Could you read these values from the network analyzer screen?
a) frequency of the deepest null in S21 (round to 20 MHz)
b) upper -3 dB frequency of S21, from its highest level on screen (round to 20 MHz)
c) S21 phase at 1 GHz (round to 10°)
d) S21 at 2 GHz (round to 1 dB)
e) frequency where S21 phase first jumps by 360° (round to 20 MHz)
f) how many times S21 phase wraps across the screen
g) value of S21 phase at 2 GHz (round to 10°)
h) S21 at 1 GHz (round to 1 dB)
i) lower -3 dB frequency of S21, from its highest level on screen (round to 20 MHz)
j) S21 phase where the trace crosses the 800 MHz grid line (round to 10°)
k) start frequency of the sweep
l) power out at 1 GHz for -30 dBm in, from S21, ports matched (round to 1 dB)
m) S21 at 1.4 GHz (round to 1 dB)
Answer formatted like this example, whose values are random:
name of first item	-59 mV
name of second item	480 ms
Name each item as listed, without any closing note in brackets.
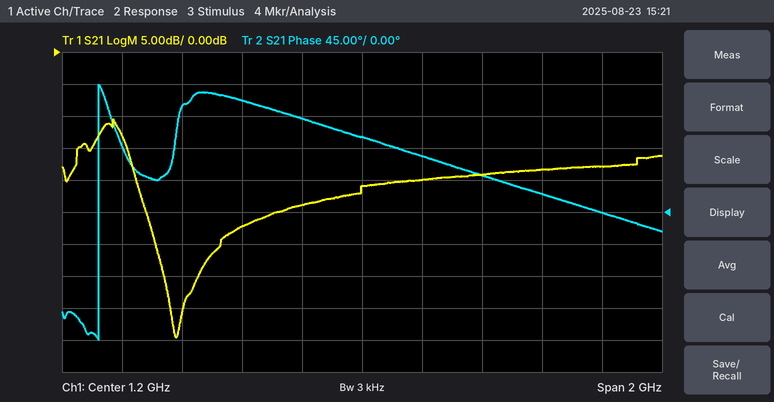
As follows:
frequency of the deepest null in S21	580 MHz
upper -3 dB frequency of S21, from its highest level on screen	400 MHz
S21 phase at 1 GHz	130°
S21 at 2 GHz	-18 dB
frequency where S21 phase first jumps by 360°	320 MHz
how many times S21 phase wraps across the screen	1
value of S21 phase at 2 GHz	0°
S21 at 1 GHz	-24 dB
lower -3 dB frequency of S21, from its highest level on screen	320 MHz
S21 phase where the trace crosses the 800 MHz grid line	160°
start frequency of the sweep	200 MHz
power out at 1 GHz for -30 dBm in, from S21, ports matched	-54 dBm
S21 at 1.4 GHz	-20 dB
